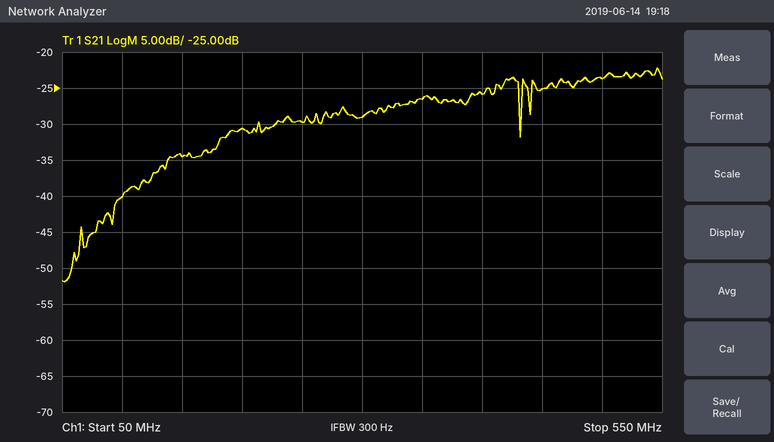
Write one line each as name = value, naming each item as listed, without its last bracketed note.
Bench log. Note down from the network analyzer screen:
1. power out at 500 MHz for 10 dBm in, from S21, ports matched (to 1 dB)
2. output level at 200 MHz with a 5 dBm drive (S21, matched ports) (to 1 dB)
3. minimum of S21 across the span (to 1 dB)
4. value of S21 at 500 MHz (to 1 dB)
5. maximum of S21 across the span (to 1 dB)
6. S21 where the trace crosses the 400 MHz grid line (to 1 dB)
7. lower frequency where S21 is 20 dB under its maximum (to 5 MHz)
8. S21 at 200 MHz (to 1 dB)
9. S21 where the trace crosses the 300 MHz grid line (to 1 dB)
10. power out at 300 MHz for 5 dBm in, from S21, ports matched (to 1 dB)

power out at 500 MHz for 10 dBm in, from S21, ports matched = -14 dBm
output level at 200 MHz with a 5 dBm drive (S21, matched ports) = -26 dBm
minimum of S21 across the span = -52 dB
value of S21 at 500 MHz = -24 dB
maximum of S21 across the span = -22 dB
S21 where the trace crosses the 400 MHz grid line = -26 dB
lower frequency where S21 is 20 dB under its maximum = 95 MHz
S21 at 200 MHz = -31 dB
S21 where the trace crosses the 300 MHz grid line = -29 dB
power out at 300 MHz for 5 dBm in, from S21, ports matched = -24 dBm
